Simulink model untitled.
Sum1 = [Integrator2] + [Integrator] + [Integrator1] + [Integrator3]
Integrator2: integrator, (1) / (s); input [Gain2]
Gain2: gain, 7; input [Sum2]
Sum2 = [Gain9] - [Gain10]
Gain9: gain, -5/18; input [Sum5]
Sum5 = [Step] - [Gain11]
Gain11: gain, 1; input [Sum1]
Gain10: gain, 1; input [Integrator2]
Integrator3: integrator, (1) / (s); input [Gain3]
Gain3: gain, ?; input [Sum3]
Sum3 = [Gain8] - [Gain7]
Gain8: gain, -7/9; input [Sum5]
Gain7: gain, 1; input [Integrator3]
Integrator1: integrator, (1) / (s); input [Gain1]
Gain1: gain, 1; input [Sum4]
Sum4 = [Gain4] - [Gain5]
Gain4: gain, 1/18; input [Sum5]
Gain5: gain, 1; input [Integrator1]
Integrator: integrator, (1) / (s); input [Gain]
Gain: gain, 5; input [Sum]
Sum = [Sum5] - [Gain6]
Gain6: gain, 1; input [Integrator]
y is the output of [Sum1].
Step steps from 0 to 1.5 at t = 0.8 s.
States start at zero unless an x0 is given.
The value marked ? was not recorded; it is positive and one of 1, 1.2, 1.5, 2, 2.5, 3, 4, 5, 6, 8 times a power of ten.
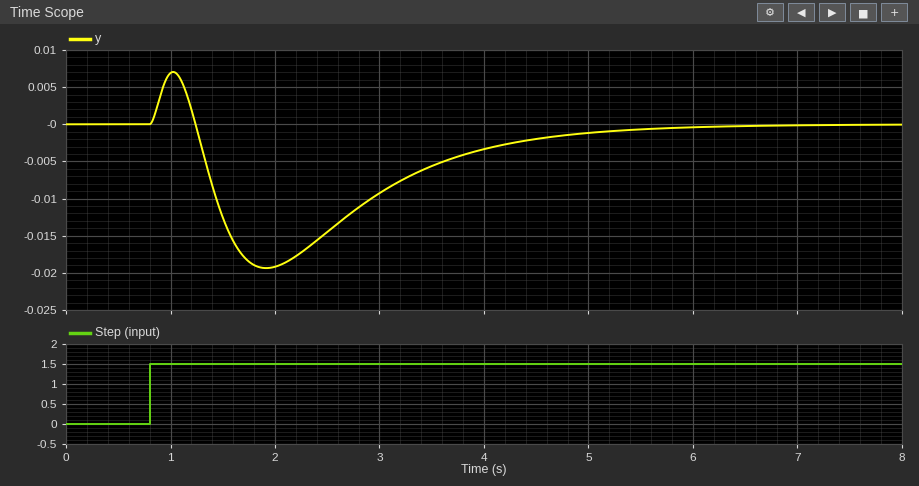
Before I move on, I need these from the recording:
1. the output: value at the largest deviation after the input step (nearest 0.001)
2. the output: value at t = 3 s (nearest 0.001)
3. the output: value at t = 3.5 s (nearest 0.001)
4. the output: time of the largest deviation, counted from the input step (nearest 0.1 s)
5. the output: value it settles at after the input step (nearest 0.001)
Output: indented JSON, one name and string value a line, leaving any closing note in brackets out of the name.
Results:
{
  "the output: value at the largest deviation after the input step": "-0.019",
  "the output: value at t = 3 s": "-0.009",
  "the output: value at t = 3.5 s": "-0.006",
  "the output: time of the largest deviation, counted from the input step": "1.1 s",
  "the output: value it settles at after the input step": "0.000"
}
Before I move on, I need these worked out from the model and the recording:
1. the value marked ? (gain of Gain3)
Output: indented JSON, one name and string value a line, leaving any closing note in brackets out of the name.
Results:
{
  "the value marked ?": "4"
}
